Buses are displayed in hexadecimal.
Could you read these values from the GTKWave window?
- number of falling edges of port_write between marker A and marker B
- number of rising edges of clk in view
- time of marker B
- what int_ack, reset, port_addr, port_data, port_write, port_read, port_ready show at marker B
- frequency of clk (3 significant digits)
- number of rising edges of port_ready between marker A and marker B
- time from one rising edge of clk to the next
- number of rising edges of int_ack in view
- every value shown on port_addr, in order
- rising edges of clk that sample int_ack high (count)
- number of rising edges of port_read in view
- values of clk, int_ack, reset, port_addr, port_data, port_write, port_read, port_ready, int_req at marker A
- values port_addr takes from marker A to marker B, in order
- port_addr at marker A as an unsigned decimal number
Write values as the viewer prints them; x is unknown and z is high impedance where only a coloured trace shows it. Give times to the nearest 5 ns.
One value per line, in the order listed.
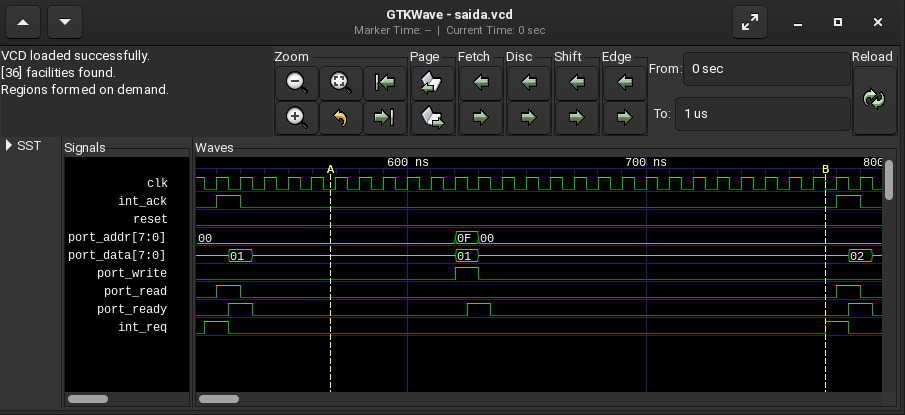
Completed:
1
28
775 ns
int_ack=0, reset=0, port_addr=00, port_data=z, port_write=0, port_read=0, port_ready=0
100 MHz
1
10 ns
2
00, 0F, 00
2
2
clk=0, int_ack=0, reset=0, port_addr=00, port_data=z, port_write=0, port_read=0, port_ready=0, int_req=0
00, 0F, 00
0
